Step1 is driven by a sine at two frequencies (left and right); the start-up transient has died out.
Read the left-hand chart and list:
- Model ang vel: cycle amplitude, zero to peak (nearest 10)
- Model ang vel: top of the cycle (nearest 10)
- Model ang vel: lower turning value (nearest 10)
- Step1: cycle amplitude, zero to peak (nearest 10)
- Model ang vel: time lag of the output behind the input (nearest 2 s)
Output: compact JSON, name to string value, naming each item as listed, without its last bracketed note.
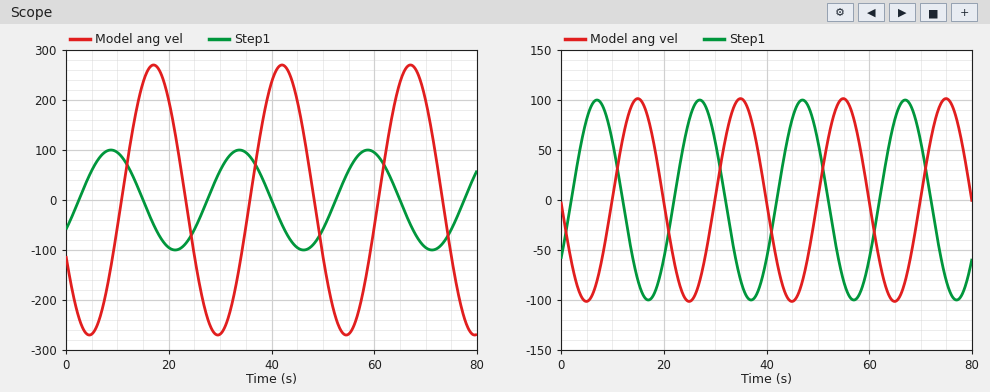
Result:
{"Model ang vel: cycle amplitude, zero to peak": "270", "Model ang vel: top of the cycle": "270", "Model ang vel: lower turning value": "-270", "Step1: cycle amplitude, zero to peak": "100", "Model ang vel: time lag of the output behind the input": "8 s"}
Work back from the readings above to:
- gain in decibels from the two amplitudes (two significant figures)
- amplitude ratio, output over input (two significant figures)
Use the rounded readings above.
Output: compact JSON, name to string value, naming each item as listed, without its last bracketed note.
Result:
{"gain in decibels from the two amplitudes": "8.6 dB", "amplitude ratio, output over input": "2.7"}
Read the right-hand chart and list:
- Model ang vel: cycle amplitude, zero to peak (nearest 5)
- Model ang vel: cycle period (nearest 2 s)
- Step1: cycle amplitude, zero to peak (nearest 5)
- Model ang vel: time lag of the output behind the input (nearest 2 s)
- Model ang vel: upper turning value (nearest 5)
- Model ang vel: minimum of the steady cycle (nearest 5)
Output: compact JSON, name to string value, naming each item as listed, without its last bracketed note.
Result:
{"Model ang vel: cycle amplitude, zero to peak": "100", "Model ang vel: cycle period": "20 s", "Step1: cycle amplitude, zero to peak": "100", "Model ang vel: time lag of the output behind the input": "8 s", "Model ang vel: upper turning value": "100", "Model ang vel: minimum of the steady cycle": "-100"}
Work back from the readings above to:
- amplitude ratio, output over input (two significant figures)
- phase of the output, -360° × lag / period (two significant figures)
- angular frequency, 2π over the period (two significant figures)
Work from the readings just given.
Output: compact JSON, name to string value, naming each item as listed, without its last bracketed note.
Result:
{"amplitude ratio, output over input": "1.0", "phase of the output, -360° × lag / period": "-140°", "angular frequency, 2π over the period": "0.31 rad/s"}
